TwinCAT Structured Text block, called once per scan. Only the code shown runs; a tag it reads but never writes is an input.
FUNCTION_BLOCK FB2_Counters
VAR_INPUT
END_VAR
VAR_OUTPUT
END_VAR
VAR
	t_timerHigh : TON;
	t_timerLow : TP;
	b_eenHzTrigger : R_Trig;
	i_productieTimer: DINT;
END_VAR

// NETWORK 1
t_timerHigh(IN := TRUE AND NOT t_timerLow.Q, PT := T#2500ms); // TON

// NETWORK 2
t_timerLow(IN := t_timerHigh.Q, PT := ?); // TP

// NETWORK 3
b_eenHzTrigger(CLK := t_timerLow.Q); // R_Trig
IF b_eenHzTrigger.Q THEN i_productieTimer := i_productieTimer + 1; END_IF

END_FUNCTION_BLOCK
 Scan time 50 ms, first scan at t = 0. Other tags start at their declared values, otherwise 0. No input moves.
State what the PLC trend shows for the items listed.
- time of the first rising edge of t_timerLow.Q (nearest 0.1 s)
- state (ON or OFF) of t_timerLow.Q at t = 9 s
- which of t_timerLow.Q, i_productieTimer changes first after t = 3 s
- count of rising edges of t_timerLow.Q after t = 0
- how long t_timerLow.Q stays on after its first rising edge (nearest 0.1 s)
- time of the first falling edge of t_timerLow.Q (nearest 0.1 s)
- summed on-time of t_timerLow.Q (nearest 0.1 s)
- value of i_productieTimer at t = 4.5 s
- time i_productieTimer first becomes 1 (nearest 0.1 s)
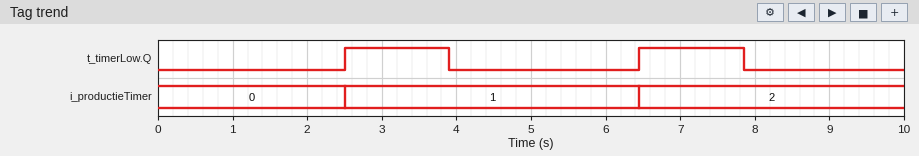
2.5 s
OFF
t_timerLow.Q
2
1.4 s
3.9 s
2.8 s
1
2.5 s
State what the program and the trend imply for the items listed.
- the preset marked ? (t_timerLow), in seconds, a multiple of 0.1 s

1.4 s
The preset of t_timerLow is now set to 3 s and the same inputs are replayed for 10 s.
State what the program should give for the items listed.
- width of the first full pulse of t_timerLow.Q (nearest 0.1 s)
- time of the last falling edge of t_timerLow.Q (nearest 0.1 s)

3.0 s
5.5 s
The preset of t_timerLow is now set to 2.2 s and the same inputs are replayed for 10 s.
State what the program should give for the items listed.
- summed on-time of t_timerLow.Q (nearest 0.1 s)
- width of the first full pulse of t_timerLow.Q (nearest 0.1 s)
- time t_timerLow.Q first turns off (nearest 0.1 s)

4.4 s
2.2 s
4.7 s
